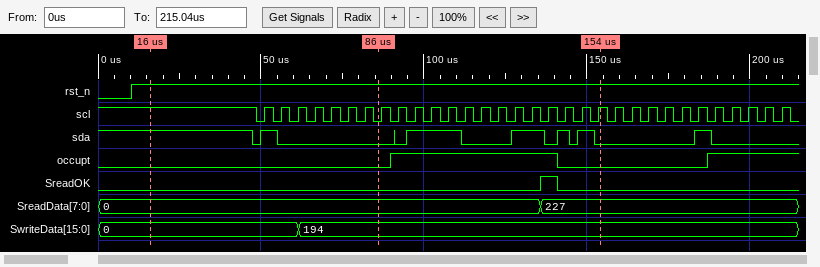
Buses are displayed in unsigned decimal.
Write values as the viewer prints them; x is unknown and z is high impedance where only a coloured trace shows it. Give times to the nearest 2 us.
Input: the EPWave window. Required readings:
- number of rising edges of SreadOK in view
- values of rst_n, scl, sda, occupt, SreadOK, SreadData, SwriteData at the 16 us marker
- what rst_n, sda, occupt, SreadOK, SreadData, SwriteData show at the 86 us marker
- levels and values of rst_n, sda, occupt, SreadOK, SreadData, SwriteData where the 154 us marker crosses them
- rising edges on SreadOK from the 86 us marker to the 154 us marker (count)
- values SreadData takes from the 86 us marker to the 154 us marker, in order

1
rst_n=1, scl=1, sda=1, occupt=0, SreadOK=0, SreadData=0, SwriteData=0
rst_n=1, sda=0, occupt=0, SreadOK=0, SreadData=0, SwriteData=194
rst_n=1, sda=0, occupt=0, SreadOK=0, SreadData=227, SwriteData=194
1
0, 227
